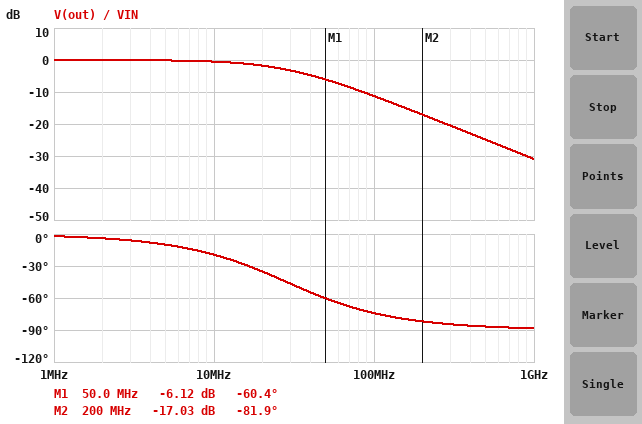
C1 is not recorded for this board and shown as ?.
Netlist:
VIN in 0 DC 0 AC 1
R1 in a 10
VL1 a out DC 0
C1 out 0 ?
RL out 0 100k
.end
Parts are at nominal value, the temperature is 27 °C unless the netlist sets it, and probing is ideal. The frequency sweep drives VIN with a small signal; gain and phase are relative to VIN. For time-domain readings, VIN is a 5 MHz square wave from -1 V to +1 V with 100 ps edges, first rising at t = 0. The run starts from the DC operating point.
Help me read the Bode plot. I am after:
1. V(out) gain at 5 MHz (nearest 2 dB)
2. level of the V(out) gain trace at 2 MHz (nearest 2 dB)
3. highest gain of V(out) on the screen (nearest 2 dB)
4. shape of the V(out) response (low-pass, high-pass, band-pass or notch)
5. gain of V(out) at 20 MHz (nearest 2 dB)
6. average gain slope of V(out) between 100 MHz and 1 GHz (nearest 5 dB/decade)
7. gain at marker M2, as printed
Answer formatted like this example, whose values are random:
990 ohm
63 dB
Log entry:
0 dB
0 dB
0 dB
low-pass
-2 dB
-20 dB/decade
-17.03 dB
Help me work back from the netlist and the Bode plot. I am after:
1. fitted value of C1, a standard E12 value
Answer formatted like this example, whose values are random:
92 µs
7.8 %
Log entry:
560 pF
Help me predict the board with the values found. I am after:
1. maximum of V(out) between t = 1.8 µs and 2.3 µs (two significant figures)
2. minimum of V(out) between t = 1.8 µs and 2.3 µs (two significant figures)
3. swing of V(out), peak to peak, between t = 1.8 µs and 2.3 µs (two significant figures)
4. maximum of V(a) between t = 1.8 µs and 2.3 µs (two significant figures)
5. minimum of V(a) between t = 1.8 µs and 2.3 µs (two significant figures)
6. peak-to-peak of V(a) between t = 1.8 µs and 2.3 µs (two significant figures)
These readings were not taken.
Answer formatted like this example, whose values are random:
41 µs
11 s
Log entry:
1.0 V
-1.0 V
2.0 V
1.0 V
-1.0 V
2.0 V
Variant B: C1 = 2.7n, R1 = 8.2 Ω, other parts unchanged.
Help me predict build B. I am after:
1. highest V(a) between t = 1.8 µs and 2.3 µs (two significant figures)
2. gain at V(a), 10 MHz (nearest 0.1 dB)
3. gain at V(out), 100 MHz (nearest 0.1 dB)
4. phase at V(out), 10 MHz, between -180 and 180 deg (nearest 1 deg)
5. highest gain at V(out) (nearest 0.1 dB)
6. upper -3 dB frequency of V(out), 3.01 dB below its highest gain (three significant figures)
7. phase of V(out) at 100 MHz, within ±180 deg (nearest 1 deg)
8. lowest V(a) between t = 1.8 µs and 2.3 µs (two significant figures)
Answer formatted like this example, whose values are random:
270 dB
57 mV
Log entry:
980 mV
-4.7 dB
-22.9 dB
-54 deg
0 dB
7.19 MHz
-86 deg
-980 mV
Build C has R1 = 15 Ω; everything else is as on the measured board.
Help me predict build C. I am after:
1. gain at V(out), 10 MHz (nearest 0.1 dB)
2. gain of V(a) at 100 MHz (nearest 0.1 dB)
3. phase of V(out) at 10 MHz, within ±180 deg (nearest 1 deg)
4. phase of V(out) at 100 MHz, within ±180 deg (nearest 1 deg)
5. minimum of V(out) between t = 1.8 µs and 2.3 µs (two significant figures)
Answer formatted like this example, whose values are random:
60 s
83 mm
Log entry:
-1.1 dB
-14.6 dB
-28 deg
-79 deg
-1.0 V
